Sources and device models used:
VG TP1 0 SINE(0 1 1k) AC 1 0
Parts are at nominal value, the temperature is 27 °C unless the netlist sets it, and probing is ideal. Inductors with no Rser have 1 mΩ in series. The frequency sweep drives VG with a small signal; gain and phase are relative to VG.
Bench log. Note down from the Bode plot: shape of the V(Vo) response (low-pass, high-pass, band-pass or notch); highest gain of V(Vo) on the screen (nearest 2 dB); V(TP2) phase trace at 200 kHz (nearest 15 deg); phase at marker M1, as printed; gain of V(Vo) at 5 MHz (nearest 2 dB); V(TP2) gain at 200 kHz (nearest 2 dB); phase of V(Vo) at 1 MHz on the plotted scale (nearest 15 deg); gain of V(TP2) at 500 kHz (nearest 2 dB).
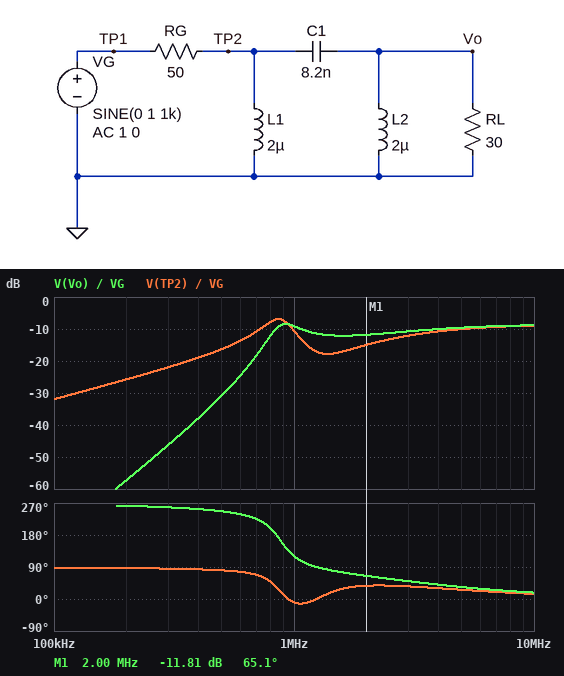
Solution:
high-pass
-8 dB
90 deg
65.1 deg
-10 dB
-26 dB
120 deg
-16 dB
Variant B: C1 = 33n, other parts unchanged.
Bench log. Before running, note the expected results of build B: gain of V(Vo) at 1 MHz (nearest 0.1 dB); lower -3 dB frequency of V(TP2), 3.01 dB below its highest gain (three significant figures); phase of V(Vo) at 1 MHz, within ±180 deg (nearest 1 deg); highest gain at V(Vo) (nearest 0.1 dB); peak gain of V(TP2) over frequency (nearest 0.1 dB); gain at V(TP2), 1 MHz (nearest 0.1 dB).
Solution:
-16.6 dB
400 kHz
76 deg
-8.5 dB
-8.0 dB
-20.6 dB
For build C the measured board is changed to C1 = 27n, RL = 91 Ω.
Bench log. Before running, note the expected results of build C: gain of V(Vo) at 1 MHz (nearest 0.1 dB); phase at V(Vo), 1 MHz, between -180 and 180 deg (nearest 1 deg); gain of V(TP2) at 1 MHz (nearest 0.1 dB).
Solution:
-15.9 dB
82 deg
-21.3 dB
